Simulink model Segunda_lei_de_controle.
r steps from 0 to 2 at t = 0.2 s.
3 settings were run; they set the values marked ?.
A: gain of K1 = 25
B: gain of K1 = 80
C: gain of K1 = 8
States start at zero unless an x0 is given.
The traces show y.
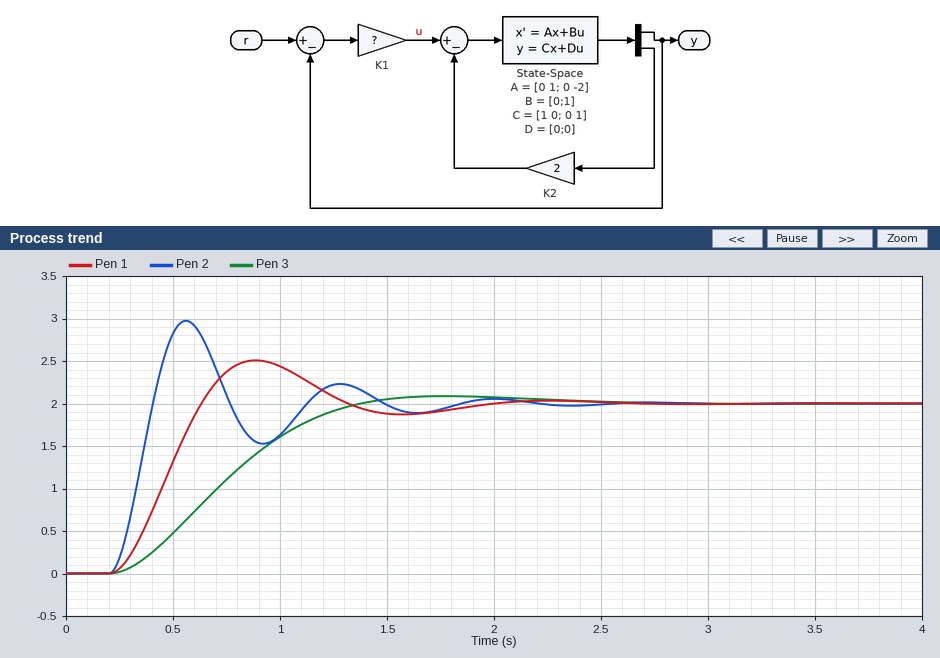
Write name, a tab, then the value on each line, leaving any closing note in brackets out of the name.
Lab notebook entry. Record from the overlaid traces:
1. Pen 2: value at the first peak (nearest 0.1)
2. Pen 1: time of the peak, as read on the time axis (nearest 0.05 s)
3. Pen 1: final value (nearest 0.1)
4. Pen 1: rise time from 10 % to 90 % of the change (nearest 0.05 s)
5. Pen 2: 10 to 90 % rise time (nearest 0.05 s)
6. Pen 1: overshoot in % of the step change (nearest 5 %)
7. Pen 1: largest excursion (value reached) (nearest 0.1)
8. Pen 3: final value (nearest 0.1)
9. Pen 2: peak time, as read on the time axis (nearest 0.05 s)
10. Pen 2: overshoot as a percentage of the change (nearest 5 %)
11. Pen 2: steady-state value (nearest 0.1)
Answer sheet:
Pen 2: value at the first peak	3.0
Pen 1: time of the peak, as read on the time axis	0.90 s
Pen 1: final value	2.0
Pen 1: rise time from 10 % to 90 % of the change	0.30 s
Pen 2: 10 to 90 % rise time	0.15 s
Pen 1: overshoot in % of the step change	25 %
Pen 1: largest excursion (value reached)	2.5
Pen 3: final value	2.0
Pen 2: peak time, as read on the time axis	0.55 s
Pen 2: overshoot as a percentage of the change	50 %
Pen 2: steady-state value	2.0
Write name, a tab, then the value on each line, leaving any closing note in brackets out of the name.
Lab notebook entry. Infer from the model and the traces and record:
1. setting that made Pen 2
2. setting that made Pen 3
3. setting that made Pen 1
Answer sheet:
setting that made Pen 2	B
setting that made Pen 3	C
setting that made Pen 1	A
